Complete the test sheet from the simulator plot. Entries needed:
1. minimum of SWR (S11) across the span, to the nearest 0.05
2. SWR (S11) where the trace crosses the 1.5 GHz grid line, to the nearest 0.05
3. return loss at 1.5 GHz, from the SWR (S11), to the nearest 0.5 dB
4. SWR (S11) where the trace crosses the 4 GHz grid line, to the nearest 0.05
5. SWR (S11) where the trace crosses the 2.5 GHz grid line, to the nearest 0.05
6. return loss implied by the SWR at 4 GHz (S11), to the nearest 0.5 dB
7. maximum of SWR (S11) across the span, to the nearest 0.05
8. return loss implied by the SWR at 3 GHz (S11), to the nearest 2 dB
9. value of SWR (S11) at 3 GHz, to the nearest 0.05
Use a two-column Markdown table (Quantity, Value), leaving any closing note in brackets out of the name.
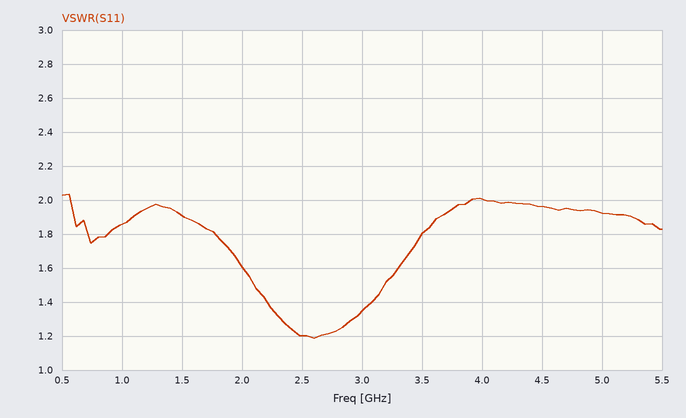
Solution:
| Quantity | Value |
|---|---|
| minimum of SWR (S11) across the span, to the nearest 0.05 | 1.20 |
| SWR (S11) where the trace crosses the 1.5 GHz grid line, to the nearest 0.05 | 1.90 |
| return loss at 1.5 GHz, from the SWR (S11), to the nearest 0.5 dB | 10.0 dB |
| SWR (S11) where the trace crosses the 4 GHz grid line, to the nearest 0.05 | 2.00 |
| SWR (S11) where the trace crosses the 2.5 GHz grid line, to the nearest 0.05 | 1.20 |
| return loss implied by the SWR at 4 GHz (S11), to the nearest 0.5 dB | 9.5 dB |
| maximum of SWR (S11) across the span, to the nearest 0.05 | 2.05 |
| return loss implied by the SWR at 3 GHz (S11), to the nearest 2 dB | 16 dB |
| value of SWR (S11) at 3 GHz, to the nearest 0.05 | 1.35 |
